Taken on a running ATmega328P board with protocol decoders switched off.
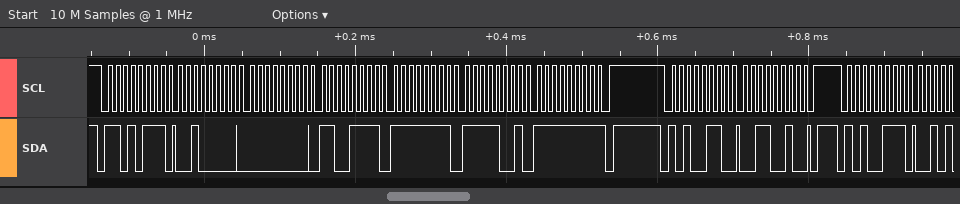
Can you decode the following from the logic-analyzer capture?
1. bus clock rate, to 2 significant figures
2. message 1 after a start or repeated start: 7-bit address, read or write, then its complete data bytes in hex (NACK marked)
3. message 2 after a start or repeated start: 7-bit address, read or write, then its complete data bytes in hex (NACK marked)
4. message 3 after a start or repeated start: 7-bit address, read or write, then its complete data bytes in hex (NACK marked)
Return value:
100 kHz
0x6B read: 20 00 CF FF F9 FF NACK
0x53 write: 32
0x53 read
